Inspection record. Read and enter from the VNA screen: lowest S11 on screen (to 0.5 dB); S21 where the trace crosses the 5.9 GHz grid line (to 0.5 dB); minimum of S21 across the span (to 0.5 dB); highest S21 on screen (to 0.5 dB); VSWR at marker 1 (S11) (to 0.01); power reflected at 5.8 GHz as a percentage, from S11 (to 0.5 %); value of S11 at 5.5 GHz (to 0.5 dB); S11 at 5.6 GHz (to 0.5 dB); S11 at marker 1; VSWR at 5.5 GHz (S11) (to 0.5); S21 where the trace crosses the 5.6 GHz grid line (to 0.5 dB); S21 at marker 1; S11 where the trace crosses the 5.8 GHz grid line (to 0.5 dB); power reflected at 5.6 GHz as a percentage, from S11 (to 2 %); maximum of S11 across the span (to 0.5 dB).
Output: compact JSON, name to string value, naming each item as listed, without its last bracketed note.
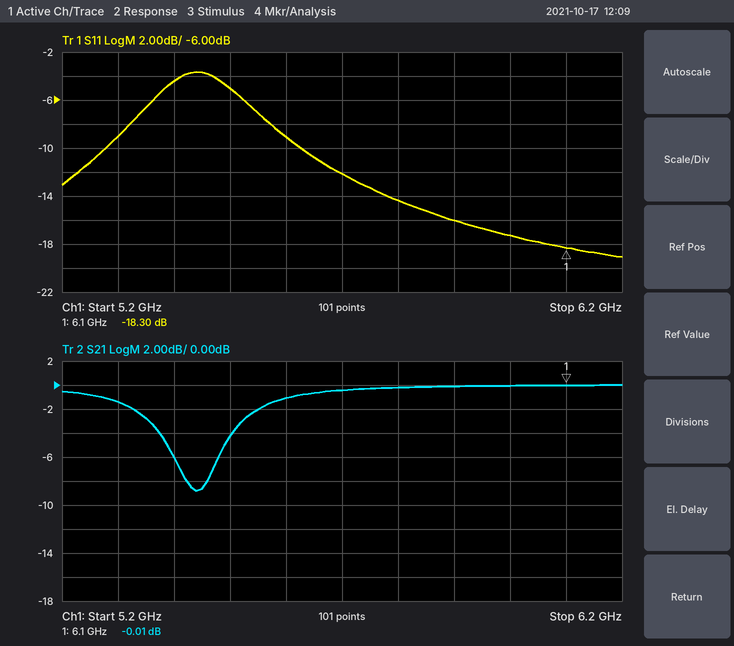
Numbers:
{"lowest S11 on screen": "-19.0 dB", "S21 where the trace crosses the 5.9 GHz grid line": "0.0 dB", "minimum of S21 across the span": "-9.0 dB", "highest S21 on screen": "0.0 dB", "VSWR at marker 1 (S11)": "1.28", "power reflected at 5.8 GHz as a percentage, from S11": "3.5 %", "value of S11 at 5.5 GHz": "-5.0 dB", "S11 at 5.6 GHz": "-9.0 dB", "S11 at marker 1": "-18.30 dB", "VSWR at 5.5 GHz (S11)": "3.5", "S21 where the trace crosses the 5.6 GHz grid line": "-1.0 dB", "S21 at marker 1": "-0.01 dB", "S11 where the trace crosses the 5.8 GHz grid line": "-14.5 dB", "power reflected at 5.6 GHz as a percentage, from S11": "12 %", "maximum of S11 across the span": "-3.5 dB"}
